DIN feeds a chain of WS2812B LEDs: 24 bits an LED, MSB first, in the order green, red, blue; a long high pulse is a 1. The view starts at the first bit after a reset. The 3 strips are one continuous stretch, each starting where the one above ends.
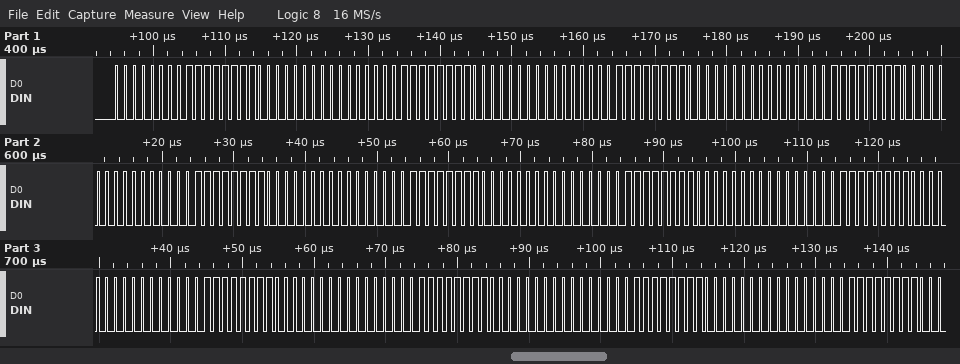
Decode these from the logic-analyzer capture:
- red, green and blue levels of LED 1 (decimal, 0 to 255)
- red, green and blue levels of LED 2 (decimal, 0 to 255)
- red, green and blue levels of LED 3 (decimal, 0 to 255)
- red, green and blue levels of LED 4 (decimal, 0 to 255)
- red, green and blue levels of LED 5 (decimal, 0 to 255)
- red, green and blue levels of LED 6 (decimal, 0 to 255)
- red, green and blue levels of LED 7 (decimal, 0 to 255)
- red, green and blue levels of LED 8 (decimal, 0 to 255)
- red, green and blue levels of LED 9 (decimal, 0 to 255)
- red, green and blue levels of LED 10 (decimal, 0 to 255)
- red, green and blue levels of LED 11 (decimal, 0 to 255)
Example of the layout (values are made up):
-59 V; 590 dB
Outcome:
255, 0, 0; 255, 0, 0; 255, 0, 0; 255, 0, 0; 255, 0, 0; 255, 0, 0; 255, 0, 0; 255, 0, 0; 255, 0, 0; 255, 0, 0; 255, 0, 0
